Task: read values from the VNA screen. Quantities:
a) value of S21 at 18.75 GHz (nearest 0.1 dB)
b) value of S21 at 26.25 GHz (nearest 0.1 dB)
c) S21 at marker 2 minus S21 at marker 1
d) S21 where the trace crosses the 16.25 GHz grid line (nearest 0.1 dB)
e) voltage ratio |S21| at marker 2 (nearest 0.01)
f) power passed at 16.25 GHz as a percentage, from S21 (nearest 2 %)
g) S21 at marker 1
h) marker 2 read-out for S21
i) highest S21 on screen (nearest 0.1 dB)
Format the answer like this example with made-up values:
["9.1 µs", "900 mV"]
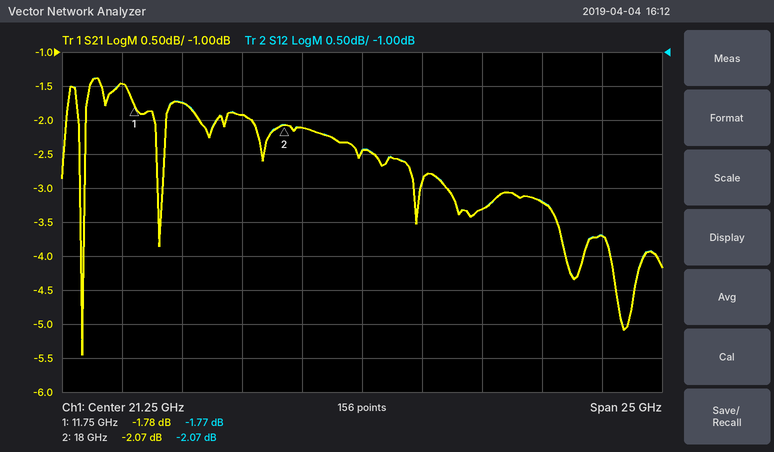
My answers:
["-2.1 dB", "-3.3 dB", "-0.29 dB", "-1.9 dB", "0.79", "64 %", "-1.78 dB", "-2.07 dB", "-1.4 dB"]
